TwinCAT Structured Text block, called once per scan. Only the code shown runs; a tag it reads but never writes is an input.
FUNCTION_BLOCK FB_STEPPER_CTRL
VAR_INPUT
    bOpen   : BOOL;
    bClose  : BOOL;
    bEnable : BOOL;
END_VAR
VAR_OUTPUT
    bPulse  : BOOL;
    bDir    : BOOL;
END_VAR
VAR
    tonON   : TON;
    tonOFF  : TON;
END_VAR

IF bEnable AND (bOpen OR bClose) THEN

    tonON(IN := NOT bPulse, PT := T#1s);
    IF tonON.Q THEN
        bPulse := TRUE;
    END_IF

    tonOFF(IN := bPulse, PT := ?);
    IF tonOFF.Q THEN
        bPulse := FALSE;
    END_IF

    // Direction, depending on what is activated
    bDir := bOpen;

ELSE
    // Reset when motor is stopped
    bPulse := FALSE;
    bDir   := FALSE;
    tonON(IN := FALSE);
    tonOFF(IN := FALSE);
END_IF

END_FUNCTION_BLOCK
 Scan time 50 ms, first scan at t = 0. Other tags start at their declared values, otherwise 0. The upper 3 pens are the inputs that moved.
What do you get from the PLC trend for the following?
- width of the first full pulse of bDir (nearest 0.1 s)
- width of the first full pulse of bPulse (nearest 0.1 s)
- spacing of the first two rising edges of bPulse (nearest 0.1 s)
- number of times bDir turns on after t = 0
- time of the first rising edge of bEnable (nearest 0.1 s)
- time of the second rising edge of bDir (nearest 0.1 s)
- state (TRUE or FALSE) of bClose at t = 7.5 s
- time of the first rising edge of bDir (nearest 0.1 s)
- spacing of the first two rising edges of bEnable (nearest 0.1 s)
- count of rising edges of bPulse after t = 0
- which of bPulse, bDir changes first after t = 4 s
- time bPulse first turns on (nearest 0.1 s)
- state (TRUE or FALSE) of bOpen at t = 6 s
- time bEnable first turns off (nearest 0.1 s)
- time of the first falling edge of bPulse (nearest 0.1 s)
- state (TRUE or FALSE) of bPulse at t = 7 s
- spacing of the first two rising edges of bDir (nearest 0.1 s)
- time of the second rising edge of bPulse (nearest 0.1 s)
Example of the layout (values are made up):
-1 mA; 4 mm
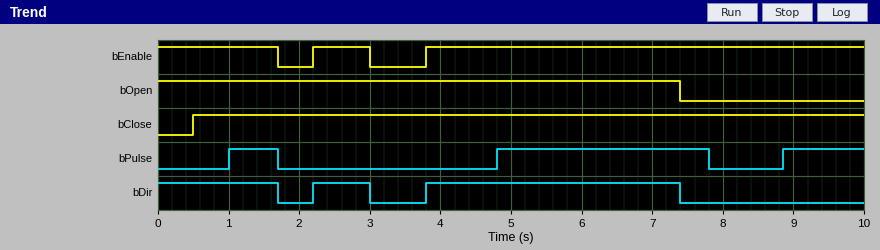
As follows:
0.8 s; 0.7 s; 3.8 s; 2; 2.2 s; 3.8 s; TRUE; 2.2 s; 1.6 s; 3; bPulse; 1.0 s; TRUE; 1.7 s; 1.7 s; TRUE; 1.6 s; 4.8 s
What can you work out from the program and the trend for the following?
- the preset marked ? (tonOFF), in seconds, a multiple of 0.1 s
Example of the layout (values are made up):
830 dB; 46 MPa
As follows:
3.0 s
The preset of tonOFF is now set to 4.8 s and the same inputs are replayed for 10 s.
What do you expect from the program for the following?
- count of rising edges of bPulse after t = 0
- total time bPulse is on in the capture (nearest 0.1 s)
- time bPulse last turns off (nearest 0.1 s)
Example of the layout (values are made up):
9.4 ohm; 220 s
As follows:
2; 5.5 s; 9.6 s
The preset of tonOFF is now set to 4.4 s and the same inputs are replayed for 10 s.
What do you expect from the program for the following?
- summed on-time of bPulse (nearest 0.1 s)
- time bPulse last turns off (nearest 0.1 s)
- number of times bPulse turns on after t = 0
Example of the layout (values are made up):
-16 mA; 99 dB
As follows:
5.1 s; 9.2 s; 2
